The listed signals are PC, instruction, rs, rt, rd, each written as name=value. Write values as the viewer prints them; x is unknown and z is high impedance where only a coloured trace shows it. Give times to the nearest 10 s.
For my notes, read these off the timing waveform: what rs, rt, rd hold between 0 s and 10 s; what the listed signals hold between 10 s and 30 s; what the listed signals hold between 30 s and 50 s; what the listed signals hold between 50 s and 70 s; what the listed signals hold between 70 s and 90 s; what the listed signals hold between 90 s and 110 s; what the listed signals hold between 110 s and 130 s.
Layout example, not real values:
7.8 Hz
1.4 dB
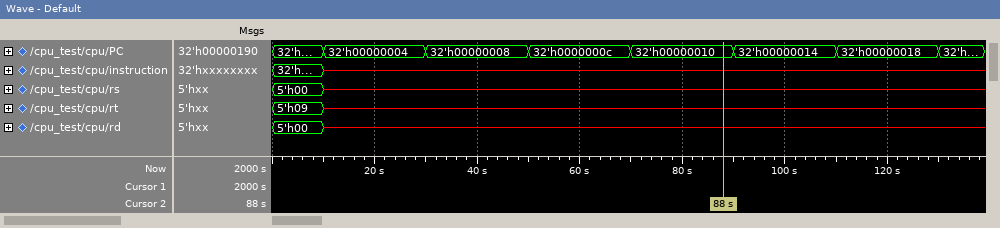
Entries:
rs=5'h00, rt=5'h09, rd=5'h00
PC=32'h00000004, instruction=x, rs=x, rt=x, rd=x
PC=32'h00000008, instruction=x, rs=x, rt=x, rd=x
PC=32'h0000000c, instruction=x, rs=x, rt=x, rd=x
PC=32'h00000010, instruction=x, rs=x, rt=x, rd=x
PC=32'h00000014, instruction=x, rs=x, rt=x, rd=x
PC=32'h00000018, instruction=x, rs=x, rt=x, rd=x
